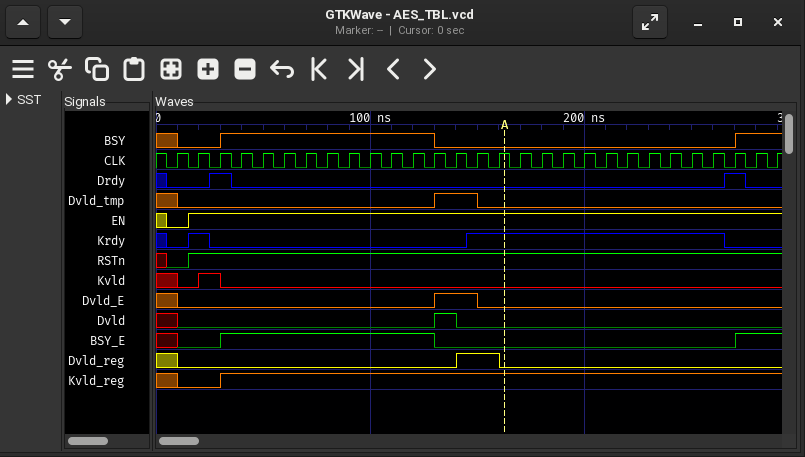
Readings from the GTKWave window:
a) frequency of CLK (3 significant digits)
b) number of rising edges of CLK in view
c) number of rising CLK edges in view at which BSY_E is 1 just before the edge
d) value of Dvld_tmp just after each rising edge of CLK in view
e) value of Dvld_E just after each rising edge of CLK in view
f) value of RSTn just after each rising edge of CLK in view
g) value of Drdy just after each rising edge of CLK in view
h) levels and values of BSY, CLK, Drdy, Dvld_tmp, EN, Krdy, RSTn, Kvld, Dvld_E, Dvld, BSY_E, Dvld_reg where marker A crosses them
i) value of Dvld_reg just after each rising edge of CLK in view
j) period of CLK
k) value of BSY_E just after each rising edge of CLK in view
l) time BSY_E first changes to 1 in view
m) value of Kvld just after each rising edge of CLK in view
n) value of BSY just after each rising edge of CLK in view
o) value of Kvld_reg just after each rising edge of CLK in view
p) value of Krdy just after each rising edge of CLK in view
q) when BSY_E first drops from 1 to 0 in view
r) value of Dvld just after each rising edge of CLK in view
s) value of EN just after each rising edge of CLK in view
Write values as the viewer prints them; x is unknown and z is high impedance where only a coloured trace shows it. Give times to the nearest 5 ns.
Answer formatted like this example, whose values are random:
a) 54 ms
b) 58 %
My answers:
a) 100 MHz
b) 29
c) 12
d) 0 0 0 0 0 0 0 0 0 0 0 0 1 1 0 0 0 0 0 0 0 0 0 0 0 0 0 0 0
e) 0 0 0 0 0 0 0 0 0 0 0 0 1 1 0 0 0 0 0 0 0 0 0 0 0 0 0 0 0
f) 0 1 1 1 1 1 1 1 1 1 1 1 1 1 1 1 1 1 1 1 1 1 1 1 1 1 1 1 1
g) 0 0 1 0 0 0 0 0 0 0 0 0 0 0 0 0 0 0 0 0 0 0 0 0 0 0 1 0 0
h) BSY=0, CLK=1, Drdy=0, Dvld_tmp=0, EN=1, Krdy=1, RSTn=1, Kvld=0, Dvld_E=0, Dvld=0, BSY_E=0, Dvld_reg=0
i) 0 0 0 0 0 0 0 0 0 0 0 0 0 1 1 0 0 0 0 0 0 0 0 0 0 0 0 0 0
j) 10 ns
k) 0 0 1 1 1 1 1 1 1 1 1 1 0 0 0 0 0 0 0 0 0 0 0 0 0 0 1 1 1
l) 30 ns
m) 0 1 0 0 0 0 0 0 0 0 0 0 0 0 0 0 0 0 0 0 0 0 0 0 0 0 0 0 0
n) 0 0 1 1 1 1 1 1 1 1 1 1 0 0 0 0 0 0 0 0 0 0 0 0 0 0 1 1 1
o) 0 0 1 1 1 1 1 1 1 1 1 1 1 1 1 1 1 1 1 1 1 1 1 1 1 1 1 1 1
p) 0 1 0 0 0 0 0 0 0 0 0 0 0 0 1 1 1 1 1 1 1 1 1 1 1 1 0 0 0
q) 130 ns
r) 0 0 0 0 0 0 0 0 0 0 0 0 1 0 0 0 0 0 0 0 0 0 0 0 0 0 0 0 0
s) 0 1 1 1 1 1 1 1 1 1 1 1 1 1 1 1 1 1 1 1 1 1 1 1 1 1 1 1 1
